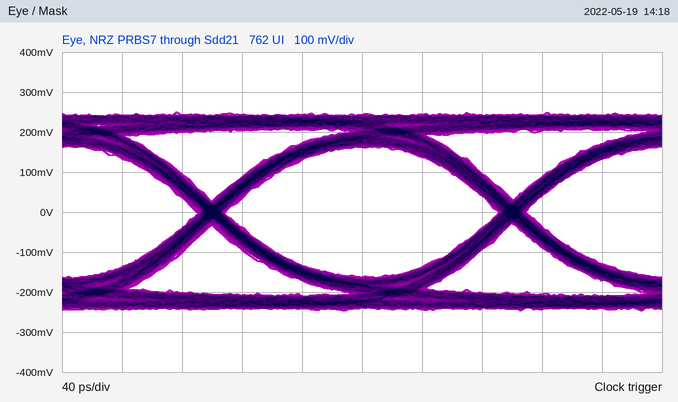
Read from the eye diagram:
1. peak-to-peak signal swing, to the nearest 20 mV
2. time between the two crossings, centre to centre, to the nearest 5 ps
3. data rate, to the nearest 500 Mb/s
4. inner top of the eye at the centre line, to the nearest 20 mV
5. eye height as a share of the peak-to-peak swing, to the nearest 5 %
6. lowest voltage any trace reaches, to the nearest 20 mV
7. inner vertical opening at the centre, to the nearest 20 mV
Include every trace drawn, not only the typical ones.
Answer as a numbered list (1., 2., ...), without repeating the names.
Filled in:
1. 500 mV
2. 200 ps
3. 5.0 Gb/s
4. 160 mV
5. 65 %
6. -240 mV
7. 320 mV
